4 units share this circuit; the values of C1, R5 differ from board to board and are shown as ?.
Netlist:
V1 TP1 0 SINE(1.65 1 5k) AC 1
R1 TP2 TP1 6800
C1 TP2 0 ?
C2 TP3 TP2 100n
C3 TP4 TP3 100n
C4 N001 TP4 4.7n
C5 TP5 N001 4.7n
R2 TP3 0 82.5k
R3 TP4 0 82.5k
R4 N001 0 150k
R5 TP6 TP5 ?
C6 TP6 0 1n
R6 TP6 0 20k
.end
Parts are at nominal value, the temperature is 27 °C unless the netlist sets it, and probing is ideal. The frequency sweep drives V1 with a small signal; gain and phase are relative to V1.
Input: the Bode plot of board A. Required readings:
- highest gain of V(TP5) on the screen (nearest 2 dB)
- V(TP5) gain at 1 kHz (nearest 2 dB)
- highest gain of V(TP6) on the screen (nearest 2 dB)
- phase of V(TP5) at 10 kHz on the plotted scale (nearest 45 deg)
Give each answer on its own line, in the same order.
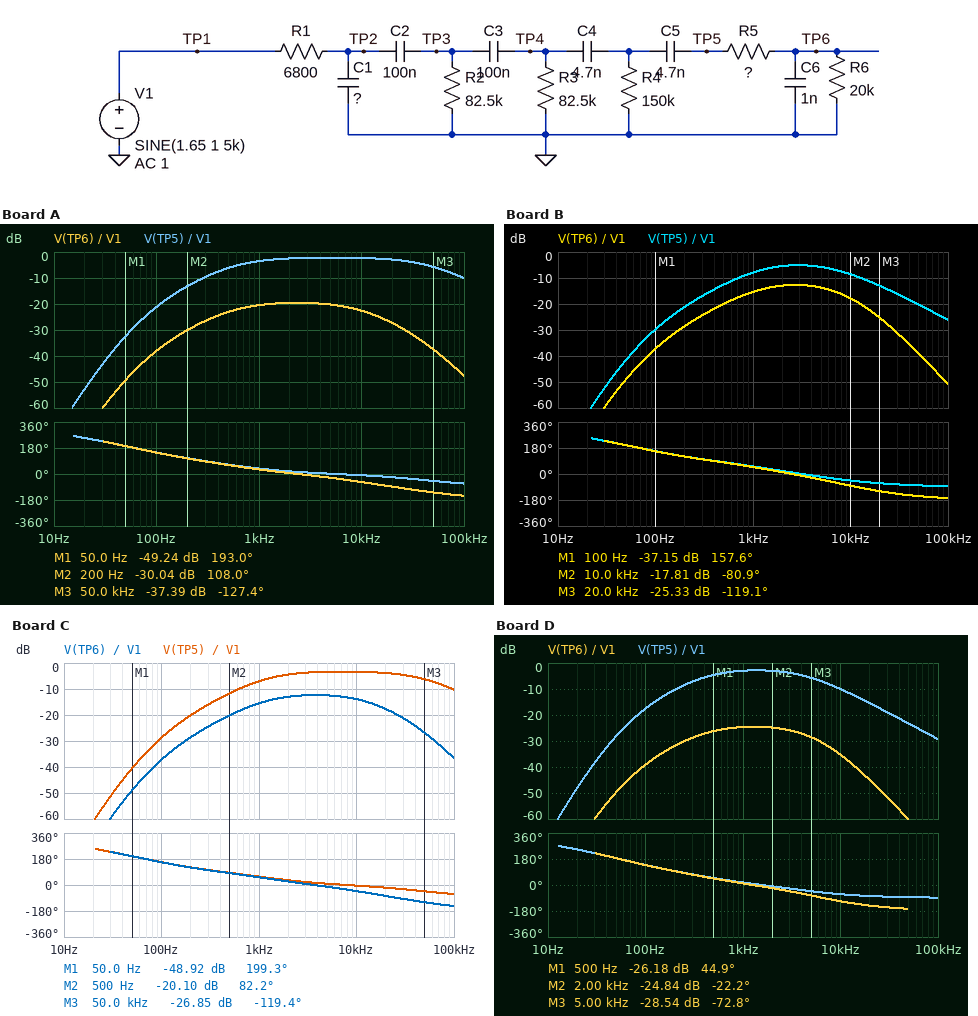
-2 dB
-4 dB
-20 dB
0 deg
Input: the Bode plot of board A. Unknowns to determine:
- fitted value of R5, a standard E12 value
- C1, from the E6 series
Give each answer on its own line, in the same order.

120 kΩ
680 pF
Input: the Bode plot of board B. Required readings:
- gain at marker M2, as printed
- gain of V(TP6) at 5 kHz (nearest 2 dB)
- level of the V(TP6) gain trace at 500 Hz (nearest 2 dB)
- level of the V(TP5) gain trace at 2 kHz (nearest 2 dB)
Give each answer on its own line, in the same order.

-17.81 dB
-14 dB
-20 dB
-6 dB
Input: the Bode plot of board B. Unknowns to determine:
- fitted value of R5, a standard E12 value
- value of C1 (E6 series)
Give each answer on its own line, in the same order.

27 kΩ
4.7 nF
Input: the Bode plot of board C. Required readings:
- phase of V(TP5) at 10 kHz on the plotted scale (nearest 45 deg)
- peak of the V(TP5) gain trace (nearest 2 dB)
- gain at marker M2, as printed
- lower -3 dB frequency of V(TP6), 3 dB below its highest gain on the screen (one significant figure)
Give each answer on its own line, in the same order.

0 deg
-4 dB
-20.10 dB
1 kHz
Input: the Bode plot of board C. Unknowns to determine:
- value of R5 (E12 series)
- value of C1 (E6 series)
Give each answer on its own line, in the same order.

33 kΩ
680 pF
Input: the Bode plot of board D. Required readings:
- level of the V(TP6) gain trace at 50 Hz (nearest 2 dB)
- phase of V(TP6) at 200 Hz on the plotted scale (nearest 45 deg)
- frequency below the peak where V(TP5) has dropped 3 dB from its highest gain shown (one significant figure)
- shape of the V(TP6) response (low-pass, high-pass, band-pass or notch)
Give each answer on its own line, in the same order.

-50 dB
90 deg
400 Hz
band-pass
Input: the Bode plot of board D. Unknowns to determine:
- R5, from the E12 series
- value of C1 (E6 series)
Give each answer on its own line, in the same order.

220 kΩ
6.8 nF
